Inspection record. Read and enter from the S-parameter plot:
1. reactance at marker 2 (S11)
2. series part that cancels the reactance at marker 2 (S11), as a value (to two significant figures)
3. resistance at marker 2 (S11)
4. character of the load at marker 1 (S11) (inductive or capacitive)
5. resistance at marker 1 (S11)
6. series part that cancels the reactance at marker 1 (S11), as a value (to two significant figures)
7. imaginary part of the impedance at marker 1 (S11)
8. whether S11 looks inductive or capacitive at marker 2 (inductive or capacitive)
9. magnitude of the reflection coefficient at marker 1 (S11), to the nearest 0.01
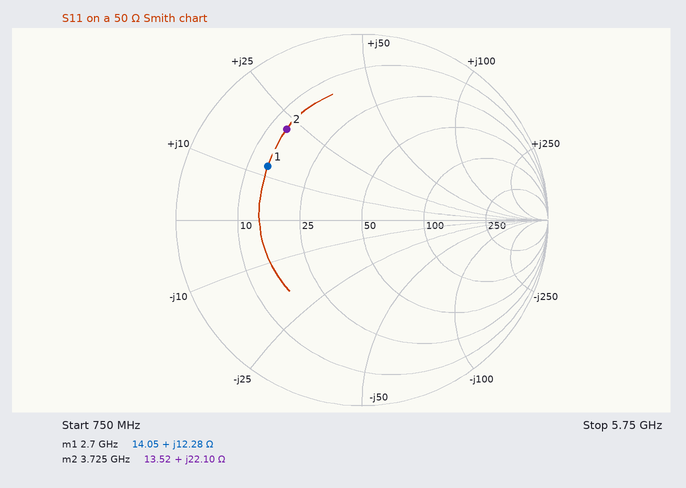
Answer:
+22.10 Ω
1.9 pF
13.52 Ω
inductive
14.05 Ω
4.8 pF
+12.28 Ω
inductive
0.58
